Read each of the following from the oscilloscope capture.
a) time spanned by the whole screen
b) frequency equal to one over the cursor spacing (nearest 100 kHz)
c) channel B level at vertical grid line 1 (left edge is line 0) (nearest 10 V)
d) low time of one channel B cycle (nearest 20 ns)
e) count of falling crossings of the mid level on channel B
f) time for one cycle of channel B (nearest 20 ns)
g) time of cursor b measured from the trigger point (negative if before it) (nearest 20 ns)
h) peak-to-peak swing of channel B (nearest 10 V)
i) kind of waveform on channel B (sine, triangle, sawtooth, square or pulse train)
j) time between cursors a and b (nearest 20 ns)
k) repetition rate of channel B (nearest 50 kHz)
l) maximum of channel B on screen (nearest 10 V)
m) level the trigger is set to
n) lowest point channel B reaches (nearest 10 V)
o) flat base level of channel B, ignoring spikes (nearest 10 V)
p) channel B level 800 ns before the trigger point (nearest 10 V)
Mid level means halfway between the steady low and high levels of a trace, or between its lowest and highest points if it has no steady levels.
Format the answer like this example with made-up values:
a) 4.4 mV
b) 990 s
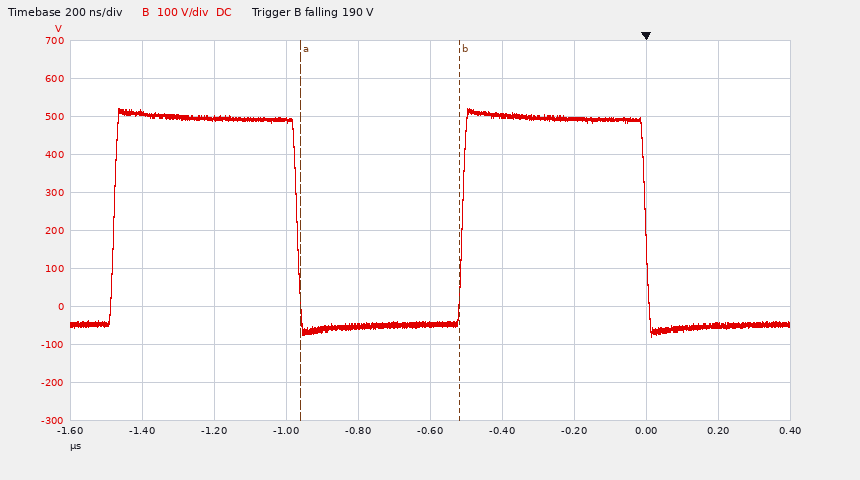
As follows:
a) 2 µs
b) 2.3 MHz
c) 510 V
d) 460 ns
e) 2
f) 960 ns
g) -520 ns
h) 600 V
i) square
j) 440 ns
k) 1.05 MHz
l) 520 V
m) 190 V
n) -80 V
o) -50 V
p) -50 V
